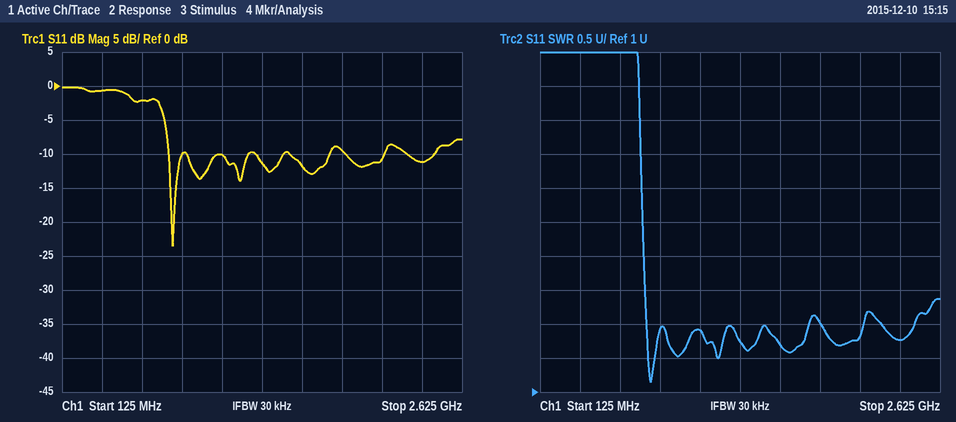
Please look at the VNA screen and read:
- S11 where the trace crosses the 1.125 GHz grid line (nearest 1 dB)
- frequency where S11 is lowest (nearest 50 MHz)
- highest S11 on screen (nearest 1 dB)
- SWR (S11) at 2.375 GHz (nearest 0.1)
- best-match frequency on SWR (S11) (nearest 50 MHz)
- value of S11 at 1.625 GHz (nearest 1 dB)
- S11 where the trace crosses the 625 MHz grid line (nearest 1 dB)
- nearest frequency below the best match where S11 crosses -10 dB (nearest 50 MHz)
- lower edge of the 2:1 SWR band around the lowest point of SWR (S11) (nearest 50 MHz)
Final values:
-10 dB
800 MHz
0 dB
1.8
800 MHz
-12 dB
-2 dB
800 MHz
800 MHz
